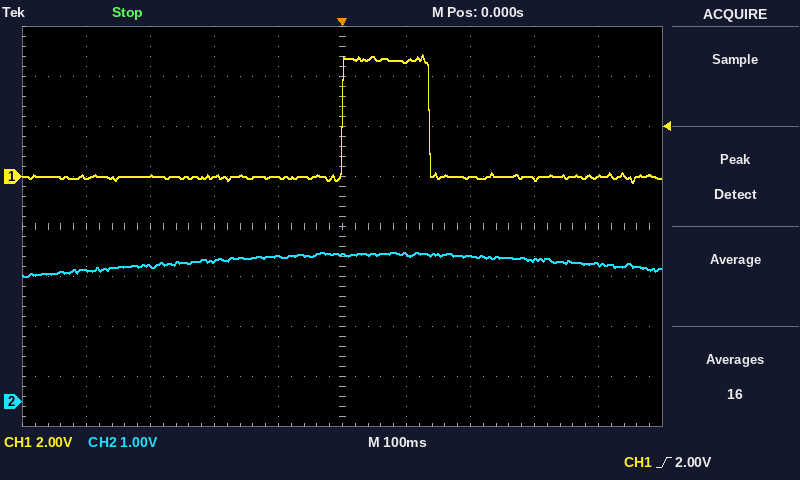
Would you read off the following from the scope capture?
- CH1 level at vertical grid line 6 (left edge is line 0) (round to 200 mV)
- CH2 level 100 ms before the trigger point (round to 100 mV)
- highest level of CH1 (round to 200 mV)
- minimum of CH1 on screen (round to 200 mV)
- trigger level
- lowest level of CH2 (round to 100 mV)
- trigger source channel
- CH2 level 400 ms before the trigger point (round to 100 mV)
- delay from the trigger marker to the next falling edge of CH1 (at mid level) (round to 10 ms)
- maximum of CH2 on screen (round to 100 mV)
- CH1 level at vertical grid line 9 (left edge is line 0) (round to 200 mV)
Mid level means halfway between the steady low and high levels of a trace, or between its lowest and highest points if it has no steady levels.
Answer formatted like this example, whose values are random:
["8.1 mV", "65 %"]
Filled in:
["4.6 V", "2.9 V", "4.8 V", "-200 mV", "2.00 V", "2.5 V", "CH1", "2.6 V", "140 ms", "3.0 V", "0.0 V"]
